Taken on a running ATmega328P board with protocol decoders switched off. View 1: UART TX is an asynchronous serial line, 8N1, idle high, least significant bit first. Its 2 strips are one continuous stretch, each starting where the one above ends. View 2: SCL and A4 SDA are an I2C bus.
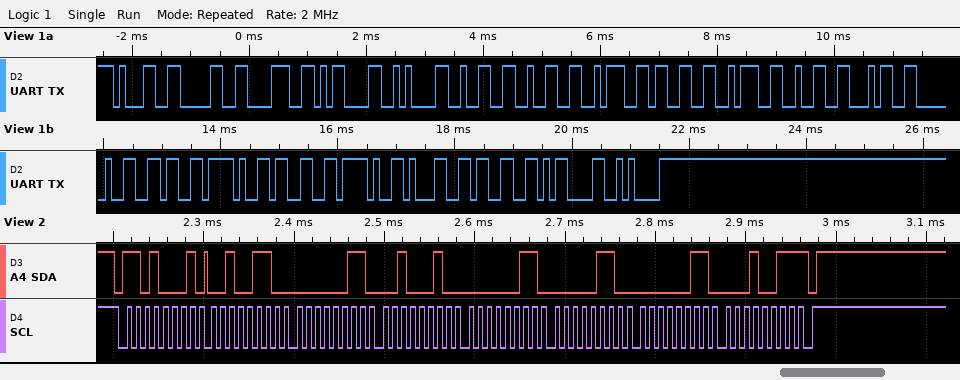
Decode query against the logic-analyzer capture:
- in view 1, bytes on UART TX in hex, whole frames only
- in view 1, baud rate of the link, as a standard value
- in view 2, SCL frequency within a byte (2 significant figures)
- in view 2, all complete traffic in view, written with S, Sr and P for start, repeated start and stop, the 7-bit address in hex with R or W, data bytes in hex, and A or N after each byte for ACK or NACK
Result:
0x31 0x30 0x38 0x0D 0x0A 0x32 0x32 0x3A 0x33 0x3A 0x32 0x34 0x20 0x36 0x2F 0x33 0x2F 0x31 0x33 0x0D 0x0A
9600 baud
100 kHz
S 68R A 26 A 03 A 22 A 03 A 06 A 03 A 13 N P
